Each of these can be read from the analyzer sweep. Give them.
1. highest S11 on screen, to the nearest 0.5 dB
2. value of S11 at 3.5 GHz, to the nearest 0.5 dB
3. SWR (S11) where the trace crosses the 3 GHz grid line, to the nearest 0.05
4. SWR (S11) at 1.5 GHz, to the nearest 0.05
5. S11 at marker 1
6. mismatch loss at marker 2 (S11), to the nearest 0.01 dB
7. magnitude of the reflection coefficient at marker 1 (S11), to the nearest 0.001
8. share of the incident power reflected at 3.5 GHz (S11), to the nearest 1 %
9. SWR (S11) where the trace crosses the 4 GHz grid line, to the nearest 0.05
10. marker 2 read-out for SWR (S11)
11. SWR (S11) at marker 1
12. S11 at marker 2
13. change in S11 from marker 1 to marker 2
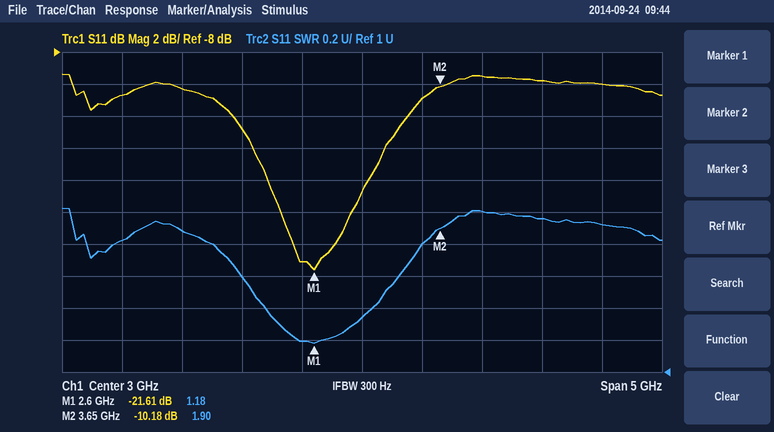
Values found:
-9.5 dB
-11.0 dB
1.35
1.90
-21.61 dB
0.44 dB
0.083
8 %
2.00
1.90
1.18
-10.18 dB
11.43 dB
